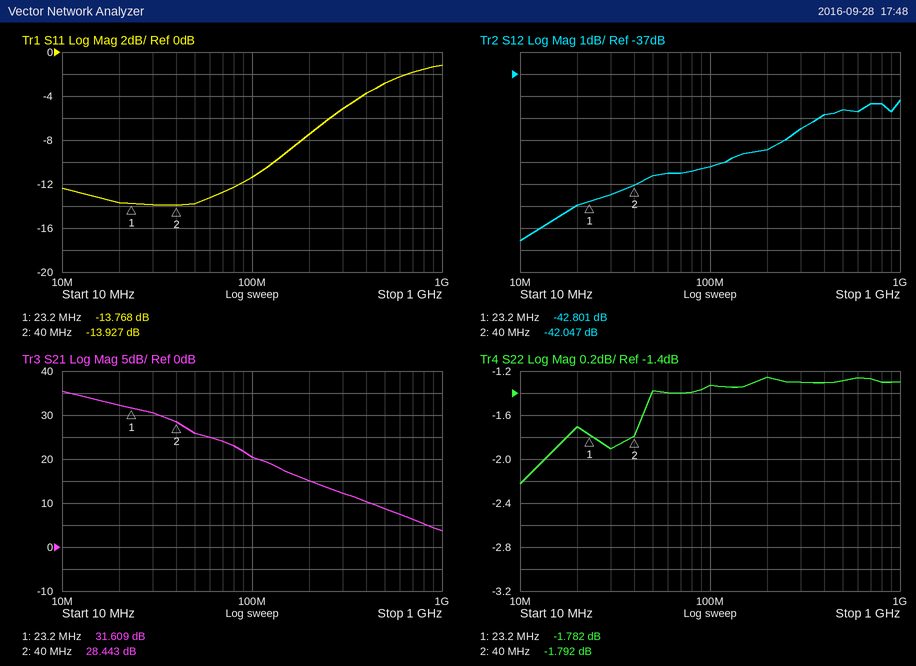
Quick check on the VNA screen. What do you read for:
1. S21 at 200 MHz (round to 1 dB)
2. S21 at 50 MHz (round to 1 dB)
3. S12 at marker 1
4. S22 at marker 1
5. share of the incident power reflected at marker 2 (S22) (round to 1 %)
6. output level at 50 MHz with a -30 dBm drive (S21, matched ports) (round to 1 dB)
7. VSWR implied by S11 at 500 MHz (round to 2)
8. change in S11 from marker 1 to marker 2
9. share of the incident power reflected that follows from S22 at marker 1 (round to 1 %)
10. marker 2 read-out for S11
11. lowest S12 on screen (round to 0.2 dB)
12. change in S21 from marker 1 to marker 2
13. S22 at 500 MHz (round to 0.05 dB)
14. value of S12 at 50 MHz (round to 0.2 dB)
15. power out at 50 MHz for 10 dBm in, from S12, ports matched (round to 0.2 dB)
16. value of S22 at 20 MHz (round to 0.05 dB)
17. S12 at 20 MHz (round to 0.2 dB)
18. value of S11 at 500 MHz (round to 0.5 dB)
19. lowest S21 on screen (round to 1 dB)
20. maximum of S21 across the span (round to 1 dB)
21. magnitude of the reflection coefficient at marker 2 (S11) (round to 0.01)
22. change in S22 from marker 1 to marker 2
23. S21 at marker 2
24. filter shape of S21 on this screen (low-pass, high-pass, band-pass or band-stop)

15 dB
26 dB
-42.801 dB
-1.782 dB
66 %
-4 dBm
6
-0.159 dB
66 %
-13.927 dB
-44.6 dB
-3.166 dB
-1.30 dB
-41.6 dB
-31.6 dBm
-1.70 dB
-43.0 dB
-3.0 dB
4 dB
35 dB
0.20
-0.010 dB
28.443 dB
low-pass
